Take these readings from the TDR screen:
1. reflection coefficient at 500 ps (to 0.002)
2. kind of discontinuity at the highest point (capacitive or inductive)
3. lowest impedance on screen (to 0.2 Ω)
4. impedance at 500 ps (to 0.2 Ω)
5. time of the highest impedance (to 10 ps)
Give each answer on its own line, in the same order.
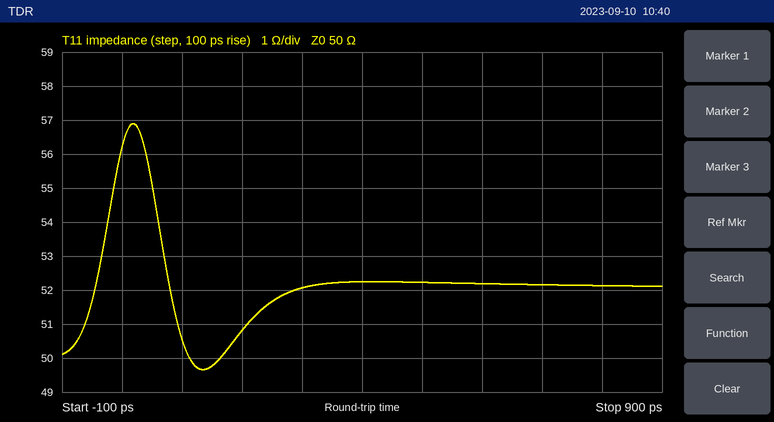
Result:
+0.022
inductive
49.6 Ω
52.2 Ω
20 ps
